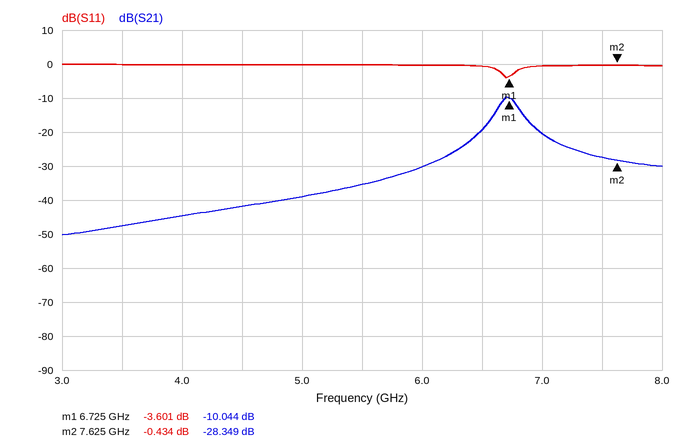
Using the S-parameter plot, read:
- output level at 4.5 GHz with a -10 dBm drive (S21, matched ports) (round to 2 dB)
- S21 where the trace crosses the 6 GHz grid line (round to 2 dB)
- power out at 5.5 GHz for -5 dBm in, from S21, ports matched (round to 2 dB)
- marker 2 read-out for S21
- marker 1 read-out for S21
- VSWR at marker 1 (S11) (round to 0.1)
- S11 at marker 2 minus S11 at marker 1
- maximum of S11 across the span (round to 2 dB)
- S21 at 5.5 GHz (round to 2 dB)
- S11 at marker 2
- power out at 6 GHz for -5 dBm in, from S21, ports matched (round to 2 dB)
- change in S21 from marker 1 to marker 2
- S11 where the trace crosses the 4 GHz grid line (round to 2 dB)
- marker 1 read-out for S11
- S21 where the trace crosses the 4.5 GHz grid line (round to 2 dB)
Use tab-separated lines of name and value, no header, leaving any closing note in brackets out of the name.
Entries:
output level at 4.5 GHz with a -10 dBm drive (S21, matched ports)	-52 dBm
S21 where the trace crosses the 6 GHz grid line	-30 dB
power out at 5.5 GHz for -5 dBm in, from S21, ports matched	-40 dBm
marker 2 read-out for S21	-28.349 dB
marker 1 read-out for S21	-10.044 dB
VSWR at marker 1 (S11)	4.9
S11 at marker 2 minus S11 at marker 1	3.167 dB
maximum of S11 across the span	0 dB
S21 at 5.5 GHz	-36 dB
S11 at marker 2	-0.434 dB
power out at 6 GHz for -5 dBm in, from S21, ports matched	-36 dBm
change in S21 from marker 1 to marker 2	-18.305 dB
S11 where the trace crosses the 4 GHz grid line	0 dB
marker 1 read-out for S11	-3.601 dB
S21 where the trace crosses the 4.5 GHz grid line	-42 dB
